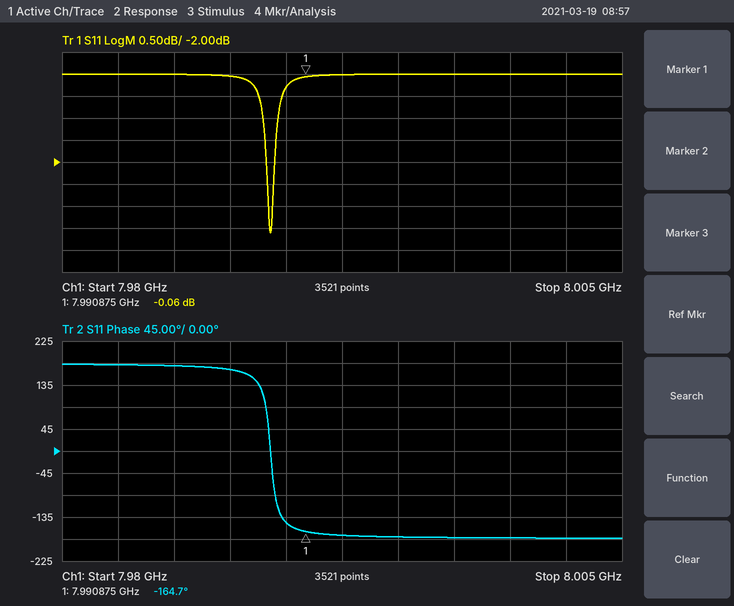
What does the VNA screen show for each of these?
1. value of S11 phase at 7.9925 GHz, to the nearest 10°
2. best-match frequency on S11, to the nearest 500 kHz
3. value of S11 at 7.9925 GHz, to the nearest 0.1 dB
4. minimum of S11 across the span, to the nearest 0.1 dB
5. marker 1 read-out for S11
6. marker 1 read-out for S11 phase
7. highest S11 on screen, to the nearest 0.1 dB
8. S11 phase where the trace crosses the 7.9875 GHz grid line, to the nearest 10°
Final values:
-170°
7.9895 GHz
0.0 dB
-3.6 dB
-0.06 dB
-164.7°
0.0 dB
170°
